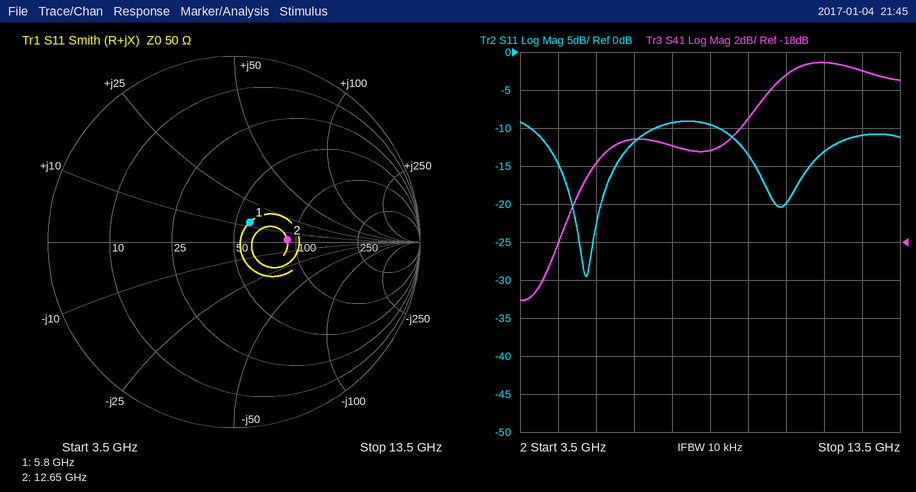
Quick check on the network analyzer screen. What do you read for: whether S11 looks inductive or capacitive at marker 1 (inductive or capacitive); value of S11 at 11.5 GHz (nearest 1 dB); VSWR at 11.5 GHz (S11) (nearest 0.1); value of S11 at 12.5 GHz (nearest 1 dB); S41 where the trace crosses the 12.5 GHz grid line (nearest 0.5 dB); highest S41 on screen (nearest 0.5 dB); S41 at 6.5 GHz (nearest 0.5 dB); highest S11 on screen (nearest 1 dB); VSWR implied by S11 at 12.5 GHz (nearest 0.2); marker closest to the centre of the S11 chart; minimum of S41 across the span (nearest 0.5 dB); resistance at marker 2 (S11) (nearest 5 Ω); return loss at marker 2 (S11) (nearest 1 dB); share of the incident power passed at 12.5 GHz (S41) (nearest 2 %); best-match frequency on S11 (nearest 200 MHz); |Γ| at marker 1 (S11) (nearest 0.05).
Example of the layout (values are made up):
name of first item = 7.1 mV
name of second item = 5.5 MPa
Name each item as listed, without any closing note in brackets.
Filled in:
whether S11 looks inductive or capacitive at marker 1 = inductive
value of S11 at 11.5 GHz = -13 dB
VSWR at 11.5 GHz (S11) = 1.6
value of S11 at 12.5 GHz = -11 dB
S41 where the trace crosses the 12.5 GHz grid line = -9.0 dB
highest S41 on screen = -8.5 dB
S41 at 6.5 GHz = -12.5 dB
highest S11 on screen = -9 dB
VSWR implied by S11 at 12.5 GHz = 1.8
marker closest to the centre of the S11 chart = marker 1
minimum of S41 across the span = -21.0 dB
resistance at marker 2 (S11) = 90 Ω
return loss at marker 2 (S11) = 11 dB
share of the incident power passed at 12.5 GHz (S41) = 12 %
best-match frequency on S11 = 5.2 GHz
|Γ| at marker 1 (S11) = 0.15
